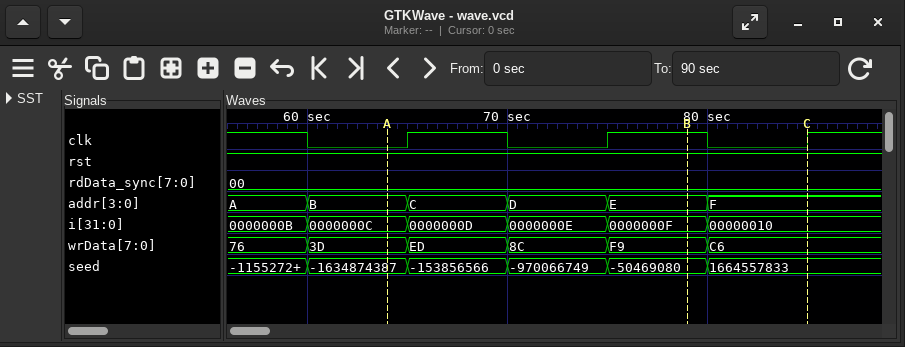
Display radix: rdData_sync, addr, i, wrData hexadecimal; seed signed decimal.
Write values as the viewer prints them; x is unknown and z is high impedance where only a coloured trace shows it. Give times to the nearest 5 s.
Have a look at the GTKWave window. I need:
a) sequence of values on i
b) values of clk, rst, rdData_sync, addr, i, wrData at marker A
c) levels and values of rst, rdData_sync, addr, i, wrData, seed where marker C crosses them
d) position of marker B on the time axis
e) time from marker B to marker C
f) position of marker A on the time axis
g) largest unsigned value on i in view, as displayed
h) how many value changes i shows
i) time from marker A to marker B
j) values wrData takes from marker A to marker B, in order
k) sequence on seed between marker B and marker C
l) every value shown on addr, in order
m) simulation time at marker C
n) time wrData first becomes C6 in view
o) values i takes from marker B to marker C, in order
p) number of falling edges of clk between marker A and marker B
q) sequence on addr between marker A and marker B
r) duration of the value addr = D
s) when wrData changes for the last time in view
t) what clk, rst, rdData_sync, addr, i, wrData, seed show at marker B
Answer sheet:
0000000B, 0000000C, 0000000D, 0000000E, 0000000F, 00000010
clk=0, rst=1, rdData_sync=00, addr=B, i=0000000C, wrData=3D
rst=1, rdData_sync=00, addr=F, i=00000010, wrData=C6, seed=1664557833
80 s
5 s
65 s
00000010
5
15 s
3D, ED, 8C, F9
-50469080, 1664557833
A, B, C, D, E, F
85 s
80 s
0000000F, 00000010
1
B, C, D, E
5 s
80 s
clk=1, rst=1, rdData_sync=00, addr=E, i=0000000F, wrData=F9, seed=-50469080
